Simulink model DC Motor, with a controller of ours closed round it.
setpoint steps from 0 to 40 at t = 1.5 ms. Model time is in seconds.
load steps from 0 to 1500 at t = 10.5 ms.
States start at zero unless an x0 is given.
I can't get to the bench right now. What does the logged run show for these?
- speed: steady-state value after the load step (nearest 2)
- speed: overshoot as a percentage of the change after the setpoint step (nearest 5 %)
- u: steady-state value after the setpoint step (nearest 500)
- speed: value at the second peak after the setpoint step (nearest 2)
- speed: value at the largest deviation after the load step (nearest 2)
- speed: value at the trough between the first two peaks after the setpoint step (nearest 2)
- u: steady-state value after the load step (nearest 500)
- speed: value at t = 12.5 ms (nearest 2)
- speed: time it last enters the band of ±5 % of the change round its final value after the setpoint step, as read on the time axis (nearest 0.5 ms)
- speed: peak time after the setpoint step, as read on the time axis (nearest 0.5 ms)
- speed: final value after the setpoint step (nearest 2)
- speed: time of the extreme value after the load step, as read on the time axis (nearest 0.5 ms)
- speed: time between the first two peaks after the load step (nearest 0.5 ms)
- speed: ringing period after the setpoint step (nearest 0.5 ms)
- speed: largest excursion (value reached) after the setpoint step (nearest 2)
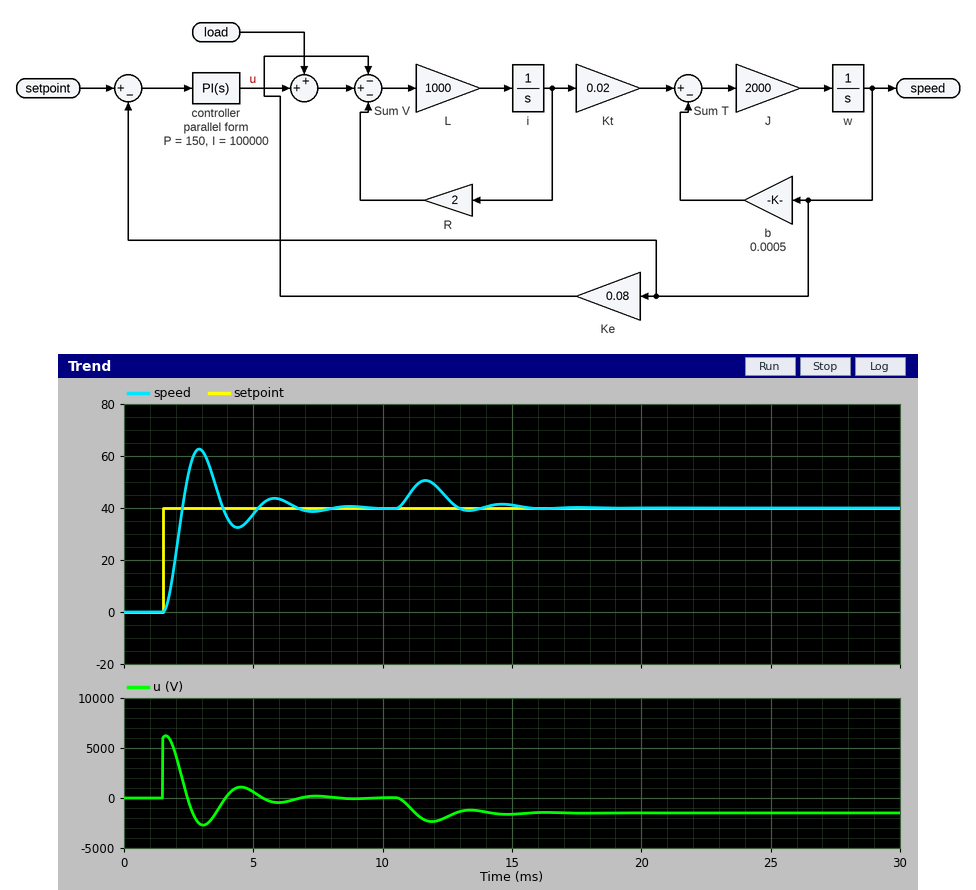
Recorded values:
40
55 %
0
44
50
32
-1500
44
6.5 ms
3.0 ms
40
11.5 ms
3.0 ms
3.0 ms
62
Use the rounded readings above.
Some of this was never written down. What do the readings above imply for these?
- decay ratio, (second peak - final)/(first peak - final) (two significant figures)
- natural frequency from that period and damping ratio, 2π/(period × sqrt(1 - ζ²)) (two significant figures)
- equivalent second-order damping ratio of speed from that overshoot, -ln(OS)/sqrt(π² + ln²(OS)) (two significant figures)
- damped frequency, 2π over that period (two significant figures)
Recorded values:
0.18
2.1 rad/ms
0.19
2.1 rad/ms
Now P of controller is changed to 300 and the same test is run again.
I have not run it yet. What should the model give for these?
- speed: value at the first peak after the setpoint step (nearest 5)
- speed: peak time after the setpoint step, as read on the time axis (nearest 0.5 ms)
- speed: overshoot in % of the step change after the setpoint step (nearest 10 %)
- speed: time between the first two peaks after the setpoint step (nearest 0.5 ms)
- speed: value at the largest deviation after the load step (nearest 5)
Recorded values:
60
2.5 ms
50 %
2.0 ms
45
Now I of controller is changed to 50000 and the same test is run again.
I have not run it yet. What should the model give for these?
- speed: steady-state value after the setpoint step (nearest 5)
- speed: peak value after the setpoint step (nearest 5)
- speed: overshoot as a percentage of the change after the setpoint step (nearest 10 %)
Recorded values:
40
55
40 %
